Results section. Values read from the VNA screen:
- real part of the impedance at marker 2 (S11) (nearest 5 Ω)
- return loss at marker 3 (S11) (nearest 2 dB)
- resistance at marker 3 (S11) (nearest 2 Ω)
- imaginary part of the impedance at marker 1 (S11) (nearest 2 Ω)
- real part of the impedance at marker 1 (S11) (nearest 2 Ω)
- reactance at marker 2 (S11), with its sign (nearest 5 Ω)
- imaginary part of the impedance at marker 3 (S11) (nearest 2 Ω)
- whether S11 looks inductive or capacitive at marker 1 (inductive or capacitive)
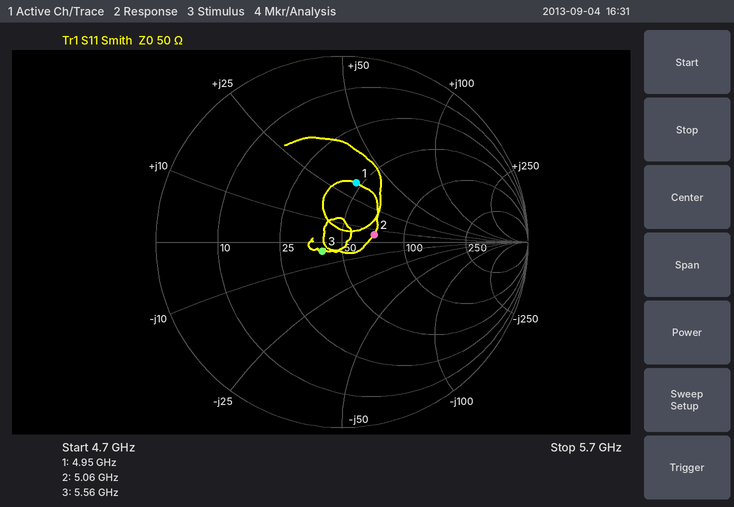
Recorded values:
70 Ω
18 dB
40 Ω
+34 Ω
46 Ω
+5 Ω
-4 Ω
inductive
